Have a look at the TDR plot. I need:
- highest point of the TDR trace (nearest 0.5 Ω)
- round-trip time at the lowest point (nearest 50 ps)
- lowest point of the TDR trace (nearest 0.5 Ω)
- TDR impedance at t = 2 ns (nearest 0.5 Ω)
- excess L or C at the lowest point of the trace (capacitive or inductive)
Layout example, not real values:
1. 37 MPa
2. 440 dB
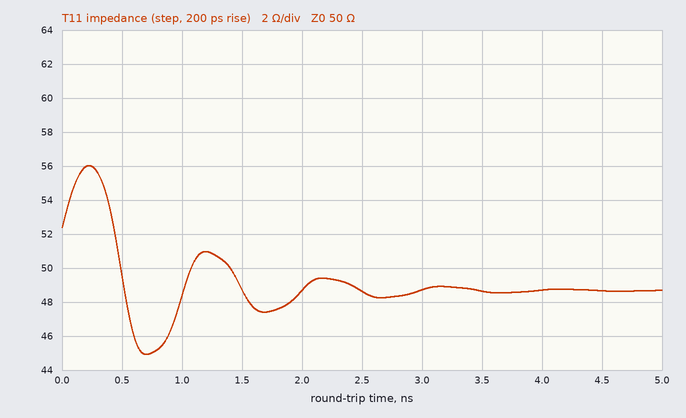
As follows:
1. 56.0 Ω
2. 700 ps
3. 45.0 Ω
4. 48.5 Ω
5. capacitive
